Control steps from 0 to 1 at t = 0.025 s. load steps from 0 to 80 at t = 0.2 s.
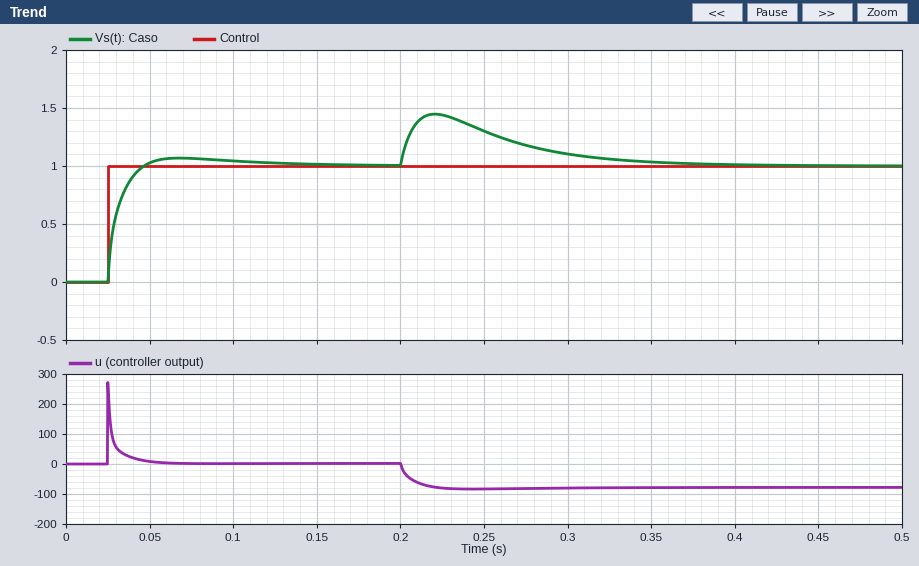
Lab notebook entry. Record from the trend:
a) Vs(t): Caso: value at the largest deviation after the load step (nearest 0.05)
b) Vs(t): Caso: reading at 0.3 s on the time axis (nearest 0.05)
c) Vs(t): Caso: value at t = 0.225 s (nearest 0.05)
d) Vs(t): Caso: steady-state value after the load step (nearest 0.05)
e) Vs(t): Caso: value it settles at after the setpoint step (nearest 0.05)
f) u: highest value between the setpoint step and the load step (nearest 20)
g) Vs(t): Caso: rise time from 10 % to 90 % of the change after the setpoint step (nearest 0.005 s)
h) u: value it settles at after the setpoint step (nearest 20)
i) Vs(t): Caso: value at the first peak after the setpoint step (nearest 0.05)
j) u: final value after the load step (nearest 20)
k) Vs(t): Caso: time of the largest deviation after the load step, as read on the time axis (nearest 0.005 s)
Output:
1.45
1.10
1.45
1.00
1.00
280
0.015 s
0
1.05
-80
0.220 s
